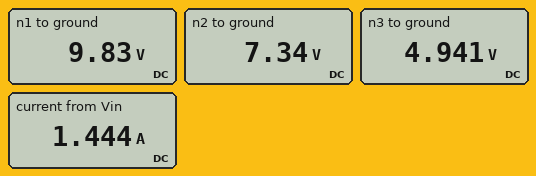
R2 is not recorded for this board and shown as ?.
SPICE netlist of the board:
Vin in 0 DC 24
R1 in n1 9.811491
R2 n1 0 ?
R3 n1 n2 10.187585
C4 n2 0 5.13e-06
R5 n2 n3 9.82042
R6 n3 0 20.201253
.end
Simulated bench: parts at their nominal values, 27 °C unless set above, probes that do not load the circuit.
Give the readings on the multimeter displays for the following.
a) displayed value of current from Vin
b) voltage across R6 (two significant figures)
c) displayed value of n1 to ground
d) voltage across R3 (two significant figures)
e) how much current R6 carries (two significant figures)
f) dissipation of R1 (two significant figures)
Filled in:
1.444 A
4.9 V
9.83 V
2.5 V
240 mA
20 W
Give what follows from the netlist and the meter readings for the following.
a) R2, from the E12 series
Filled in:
8.2 Ω
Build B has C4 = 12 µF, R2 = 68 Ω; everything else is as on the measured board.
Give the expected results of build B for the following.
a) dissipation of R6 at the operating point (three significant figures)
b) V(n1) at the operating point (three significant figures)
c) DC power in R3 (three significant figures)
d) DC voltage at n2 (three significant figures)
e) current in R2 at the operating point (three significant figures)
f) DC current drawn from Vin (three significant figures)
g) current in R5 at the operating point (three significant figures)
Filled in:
3.73 W
17.3 V
1.88 W
12.9 V
254 mA
684 mA
430 mA
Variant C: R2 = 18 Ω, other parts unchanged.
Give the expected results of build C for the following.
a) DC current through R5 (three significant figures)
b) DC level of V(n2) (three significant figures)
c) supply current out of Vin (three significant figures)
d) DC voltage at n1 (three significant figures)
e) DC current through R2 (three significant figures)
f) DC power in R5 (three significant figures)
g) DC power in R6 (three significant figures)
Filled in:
334 mA
10.0 V
1.08 A
13.4 V
745 mA
1.09 W
2.25 W
